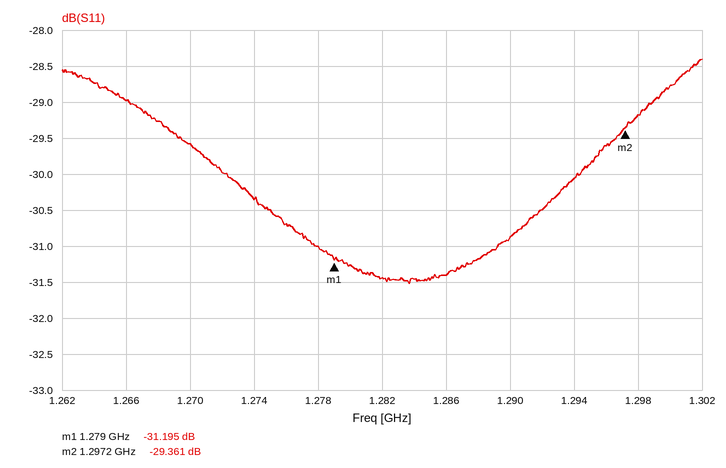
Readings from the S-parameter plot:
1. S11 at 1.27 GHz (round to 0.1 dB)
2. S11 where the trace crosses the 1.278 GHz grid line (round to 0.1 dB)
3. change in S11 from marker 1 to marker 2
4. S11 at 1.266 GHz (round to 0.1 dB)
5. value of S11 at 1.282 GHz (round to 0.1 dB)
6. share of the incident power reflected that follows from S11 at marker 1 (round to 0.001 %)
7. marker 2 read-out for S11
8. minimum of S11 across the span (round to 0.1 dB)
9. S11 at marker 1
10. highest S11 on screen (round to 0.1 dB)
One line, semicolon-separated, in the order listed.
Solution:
-29.6 dB; -31.0 dB; 1.834 dB; -29.0 dB; -31.4 dB; 0.076 %; -29.361 dB; -31.5 dB; -31.195 dB; -28.4 dB
